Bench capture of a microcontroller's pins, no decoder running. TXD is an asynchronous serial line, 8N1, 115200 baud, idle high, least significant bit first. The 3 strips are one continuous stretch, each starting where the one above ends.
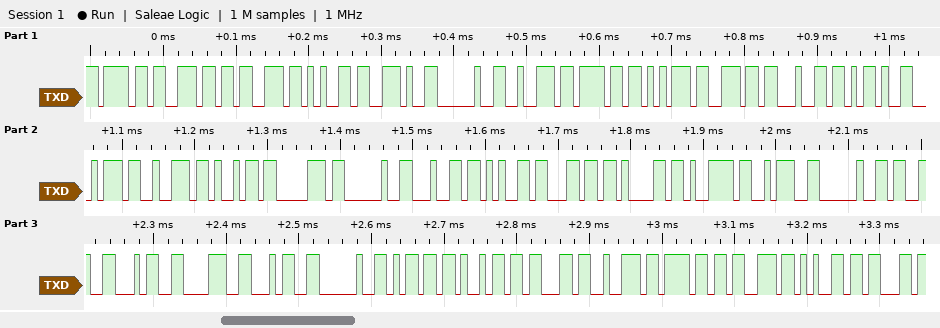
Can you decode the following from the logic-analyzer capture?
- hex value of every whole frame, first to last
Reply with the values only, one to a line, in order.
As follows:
6F 6E 73 65 2E 20 72 6F 75 6E 64 2D 74 72 69 70 20 64 65 6C 61 79 3A 20 33 34 38 34 20 6D 69 63 72 6F 73 65 63
